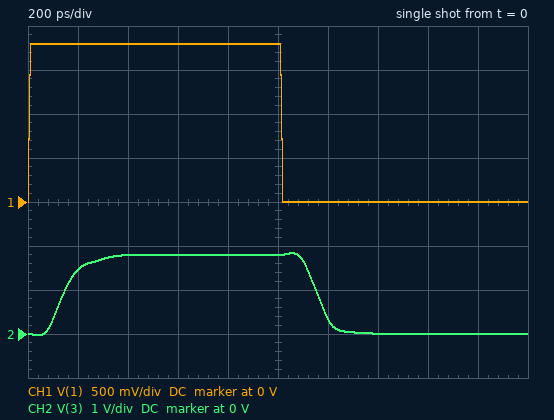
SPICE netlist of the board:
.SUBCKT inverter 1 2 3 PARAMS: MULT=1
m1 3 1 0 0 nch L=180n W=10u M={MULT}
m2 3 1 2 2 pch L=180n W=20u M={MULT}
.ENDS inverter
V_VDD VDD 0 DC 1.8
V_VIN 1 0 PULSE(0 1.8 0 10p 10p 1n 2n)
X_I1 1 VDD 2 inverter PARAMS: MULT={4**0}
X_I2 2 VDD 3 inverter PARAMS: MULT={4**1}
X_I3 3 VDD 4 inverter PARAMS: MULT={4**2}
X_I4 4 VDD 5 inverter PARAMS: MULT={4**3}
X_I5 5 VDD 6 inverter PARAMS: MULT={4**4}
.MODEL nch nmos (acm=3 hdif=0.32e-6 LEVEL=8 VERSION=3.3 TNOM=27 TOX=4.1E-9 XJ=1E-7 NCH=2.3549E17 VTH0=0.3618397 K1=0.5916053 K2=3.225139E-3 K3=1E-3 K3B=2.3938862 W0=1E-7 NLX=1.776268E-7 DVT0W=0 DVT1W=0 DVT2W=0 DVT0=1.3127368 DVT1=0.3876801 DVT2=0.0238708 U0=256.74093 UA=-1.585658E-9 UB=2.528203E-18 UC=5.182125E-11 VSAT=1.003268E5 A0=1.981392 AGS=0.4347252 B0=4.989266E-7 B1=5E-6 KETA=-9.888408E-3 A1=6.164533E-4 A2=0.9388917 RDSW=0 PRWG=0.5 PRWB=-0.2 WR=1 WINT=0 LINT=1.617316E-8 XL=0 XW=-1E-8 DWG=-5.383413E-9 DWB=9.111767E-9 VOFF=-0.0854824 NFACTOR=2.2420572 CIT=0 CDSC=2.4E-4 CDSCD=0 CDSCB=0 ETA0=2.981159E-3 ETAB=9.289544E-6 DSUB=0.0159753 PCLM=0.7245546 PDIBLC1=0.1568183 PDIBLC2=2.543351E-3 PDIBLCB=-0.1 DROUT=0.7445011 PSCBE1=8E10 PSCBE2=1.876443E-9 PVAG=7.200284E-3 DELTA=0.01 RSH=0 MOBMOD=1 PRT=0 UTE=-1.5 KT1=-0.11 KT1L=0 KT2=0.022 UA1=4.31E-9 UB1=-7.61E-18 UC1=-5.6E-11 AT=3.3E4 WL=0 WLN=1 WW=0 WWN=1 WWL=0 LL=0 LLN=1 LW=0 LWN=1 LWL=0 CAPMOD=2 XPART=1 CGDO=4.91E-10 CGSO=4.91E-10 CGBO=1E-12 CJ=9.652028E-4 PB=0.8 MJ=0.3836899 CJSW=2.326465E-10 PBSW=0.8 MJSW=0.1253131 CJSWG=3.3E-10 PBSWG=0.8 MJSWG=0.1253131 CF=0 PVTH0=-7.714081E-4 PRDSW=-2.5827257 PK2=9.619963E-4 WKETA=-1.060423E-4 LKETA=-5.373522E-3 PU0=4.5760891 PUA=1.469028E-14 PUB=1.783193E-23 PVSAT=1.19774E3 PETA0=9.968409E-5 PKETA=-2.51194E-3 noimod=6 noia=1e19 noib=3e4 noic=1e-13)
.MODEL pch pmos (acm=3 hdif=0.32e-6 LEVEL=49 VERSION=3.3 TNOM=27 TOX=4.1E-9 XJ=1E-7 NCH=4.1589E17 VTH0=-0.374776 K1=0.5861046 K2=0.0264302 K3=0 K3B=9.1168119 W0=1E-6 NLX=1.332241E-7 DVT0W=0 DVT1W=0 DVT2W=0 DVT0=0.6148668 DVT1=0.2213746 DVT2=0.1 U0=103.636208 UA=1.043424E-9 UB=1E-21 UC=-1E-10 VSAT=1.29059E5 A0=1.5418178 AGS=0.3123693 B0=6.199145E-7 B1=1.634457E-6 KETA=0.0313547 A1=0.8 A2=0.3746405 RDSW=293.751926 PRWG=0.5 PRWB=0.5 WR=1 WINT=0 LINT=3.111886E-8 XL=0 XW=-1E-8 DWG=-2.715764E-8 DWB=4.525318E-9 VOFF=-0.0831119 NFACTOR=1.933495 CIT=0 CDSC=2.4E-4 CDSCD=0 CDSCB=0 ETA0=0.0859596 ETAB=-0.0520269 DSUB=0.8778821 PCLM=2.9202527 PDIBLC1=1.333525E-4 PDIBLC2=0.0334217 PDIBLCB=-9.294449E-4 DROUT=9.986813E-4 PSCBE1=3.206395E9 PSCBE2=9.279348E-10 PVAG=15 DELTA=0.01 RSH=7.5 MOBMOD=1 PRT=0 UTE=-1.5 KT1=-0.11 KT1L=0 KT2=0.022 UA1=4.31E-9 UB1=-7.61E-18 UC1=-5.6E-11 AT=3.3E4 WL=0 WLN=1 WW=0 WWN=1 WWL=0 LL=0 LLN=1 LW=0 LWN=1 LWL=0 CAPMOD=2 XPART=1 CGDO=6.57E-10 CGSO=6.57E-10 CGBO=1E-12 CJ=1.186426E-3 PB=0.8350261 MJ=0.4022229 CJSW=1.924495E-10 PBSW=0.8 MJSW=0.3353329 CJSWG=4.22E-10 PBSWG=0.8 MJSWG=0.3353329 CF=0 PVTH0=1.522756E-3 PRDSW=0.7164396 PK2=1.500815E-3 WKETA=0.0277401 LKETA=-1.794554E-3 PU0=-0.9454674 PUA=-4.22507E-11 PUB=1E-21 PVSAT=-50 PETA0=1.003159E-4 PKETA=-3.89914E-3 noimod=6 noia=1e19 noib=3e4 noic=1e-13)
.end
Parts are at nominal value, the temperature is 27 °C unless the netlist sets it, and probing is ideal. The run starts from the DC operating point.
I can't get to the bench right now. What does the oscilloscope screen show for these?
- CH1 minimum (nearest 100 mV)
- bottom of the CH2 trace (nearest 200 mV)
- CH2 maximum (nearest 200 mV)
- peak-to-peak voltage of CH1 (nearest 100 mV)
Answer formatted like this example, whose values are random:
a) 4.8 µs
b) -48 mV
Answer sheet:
a) 0 V
b) 0 V
c) 1.8 V
d) 1.8 V
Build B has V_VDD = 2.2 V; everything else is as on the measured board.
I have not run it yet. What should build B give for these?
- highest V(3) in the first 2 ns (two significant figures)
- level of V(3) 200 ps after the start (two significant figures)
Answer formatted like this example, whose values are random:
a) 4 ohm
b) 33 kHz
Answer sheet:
a) 2.2 V
b) 1.8 V
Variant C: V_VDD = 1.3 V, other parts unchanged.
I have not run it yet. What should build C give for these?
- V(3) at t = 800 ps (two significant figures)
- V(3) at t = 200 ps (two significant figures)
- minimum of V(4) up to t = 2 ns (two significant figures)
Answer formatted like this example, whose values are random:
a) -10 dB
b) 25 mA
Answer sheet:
a) 1.3 V
b) 910 mV
c) -20 mV
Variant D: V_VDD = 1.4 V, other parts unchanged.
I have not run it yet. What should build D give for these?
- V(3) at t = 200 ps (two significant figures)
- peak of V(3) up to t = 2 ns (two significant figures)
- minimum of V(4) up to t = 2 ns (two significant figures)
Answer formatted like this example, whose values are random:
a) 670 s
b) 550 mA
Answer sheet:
a) 1.0 V
b) 1.4 V
c) -19 mV
